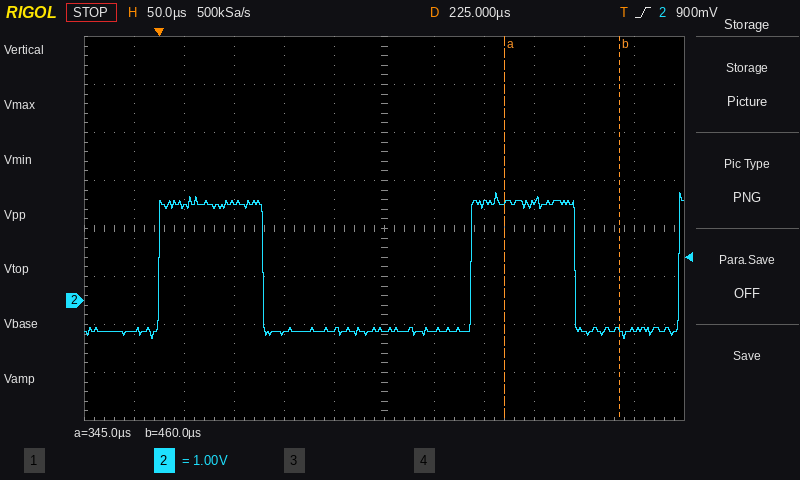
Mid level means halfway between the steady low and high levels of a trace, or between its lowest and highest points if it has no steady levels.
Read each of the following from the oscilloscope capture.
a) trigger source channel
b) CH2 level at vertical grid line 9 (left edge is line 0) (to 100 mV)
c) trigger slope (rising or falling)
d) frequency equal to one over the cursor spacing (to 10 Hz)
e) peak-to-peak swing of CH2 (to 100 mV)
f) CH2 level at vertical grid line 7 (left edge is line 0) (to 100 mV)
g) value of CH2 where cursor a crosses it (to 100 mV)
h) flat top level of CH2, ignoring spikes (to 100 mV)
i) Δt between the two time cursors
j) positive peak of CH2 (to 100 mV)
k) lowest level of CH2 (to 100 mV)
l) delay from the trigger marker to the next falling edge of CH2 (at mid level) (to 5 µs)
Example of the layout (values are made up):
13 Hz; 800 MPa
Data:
CH2; 2.1 V; rising; 8.70 kHz; 3.0 V; -600 mV; 2.0 V; 2.0 V; 115 µs; 2.2 V; -800 mV; 105 µs
